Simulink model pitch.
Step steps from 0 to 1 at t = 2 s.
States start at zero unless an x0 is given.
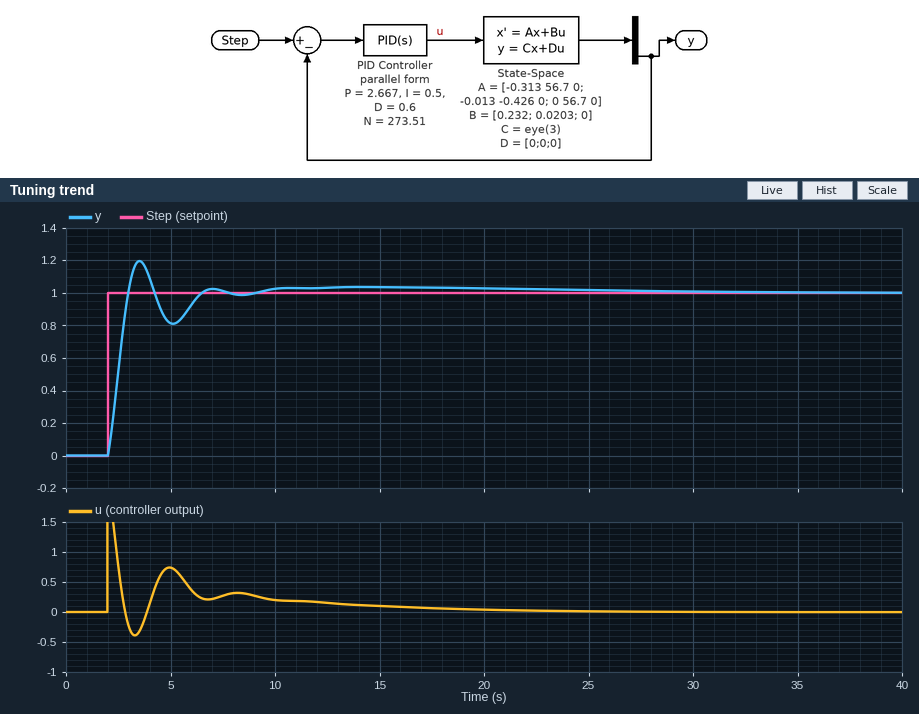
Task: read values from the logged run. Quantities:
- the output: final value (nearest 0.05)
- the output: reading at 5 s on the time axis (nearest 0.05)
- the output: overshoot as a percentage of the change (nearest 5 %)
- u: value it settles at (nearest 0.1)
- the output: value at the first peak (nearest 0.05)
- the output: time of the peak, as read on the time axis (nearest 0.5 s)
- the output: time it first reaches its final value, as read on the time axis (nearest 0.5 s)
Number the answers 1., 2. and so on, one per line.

1. 1.00
2. 0.80
3. 20 %
4. 0.0
5. 1.20
6. 3.5 s
7. 3.0 s
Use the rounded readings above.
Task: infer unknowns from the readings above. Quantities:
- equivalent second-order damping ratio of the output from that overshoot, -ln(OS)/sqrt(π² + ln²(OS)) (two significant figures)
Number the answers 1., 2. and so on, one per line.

1. 0.46
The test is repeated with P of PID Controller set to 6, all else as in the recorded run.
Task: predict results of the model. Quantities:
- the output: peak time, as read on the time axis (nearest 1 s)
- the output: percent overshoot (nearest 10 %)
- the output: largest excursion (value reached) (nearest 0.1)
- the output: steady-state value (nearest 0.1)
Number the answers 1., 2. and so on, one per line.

1. 3 s
2. 40 %
3. 1.4
4. 1.0
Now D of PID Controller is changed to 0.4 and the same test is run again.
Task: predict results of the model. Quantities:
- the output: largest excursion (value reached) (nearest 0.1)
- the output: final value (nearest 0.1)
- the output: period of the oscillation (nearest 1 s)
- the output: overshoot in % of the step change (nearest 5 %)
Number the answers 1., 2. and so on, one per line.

1. 1.3
2. 1.0
3. 3 s
4. 25 %
